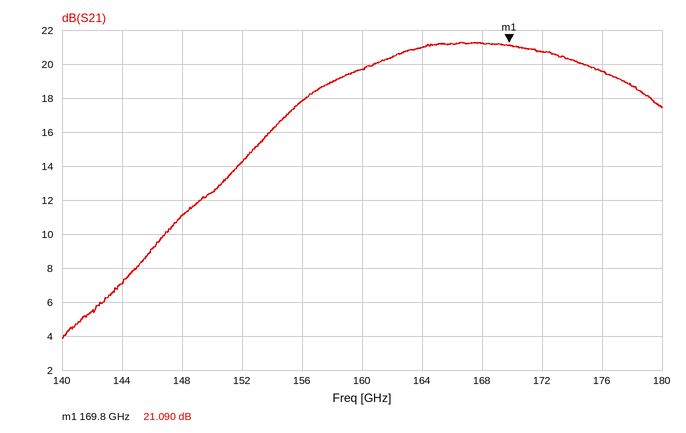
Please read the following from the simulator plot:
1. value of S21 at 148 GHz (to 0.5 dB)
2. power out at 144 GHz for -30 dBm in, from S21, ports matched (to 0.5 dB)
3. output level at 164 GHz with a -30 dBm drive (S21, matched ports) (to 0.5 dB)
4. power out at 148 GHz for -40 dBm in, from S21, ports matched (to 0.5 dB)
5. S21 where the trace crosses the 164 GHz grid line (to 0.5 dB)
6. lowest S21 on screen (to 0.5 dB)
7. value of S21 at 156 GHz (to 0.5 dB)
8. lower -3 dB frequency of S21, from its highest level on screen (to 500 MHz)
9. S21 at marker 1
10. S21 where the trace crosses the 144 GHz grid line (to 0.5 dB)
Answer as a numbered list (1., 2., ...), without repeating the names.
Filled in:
1. 11.0 dB
2. -23.0 dBm
3. -9.0 dBm
4. -29.0 dBm
5. 21.0 dB
6. 4.0 dB
7. 18.0 dB
8. 156.5 GHz
9. 21.090 dB
10. 7.0 dB
